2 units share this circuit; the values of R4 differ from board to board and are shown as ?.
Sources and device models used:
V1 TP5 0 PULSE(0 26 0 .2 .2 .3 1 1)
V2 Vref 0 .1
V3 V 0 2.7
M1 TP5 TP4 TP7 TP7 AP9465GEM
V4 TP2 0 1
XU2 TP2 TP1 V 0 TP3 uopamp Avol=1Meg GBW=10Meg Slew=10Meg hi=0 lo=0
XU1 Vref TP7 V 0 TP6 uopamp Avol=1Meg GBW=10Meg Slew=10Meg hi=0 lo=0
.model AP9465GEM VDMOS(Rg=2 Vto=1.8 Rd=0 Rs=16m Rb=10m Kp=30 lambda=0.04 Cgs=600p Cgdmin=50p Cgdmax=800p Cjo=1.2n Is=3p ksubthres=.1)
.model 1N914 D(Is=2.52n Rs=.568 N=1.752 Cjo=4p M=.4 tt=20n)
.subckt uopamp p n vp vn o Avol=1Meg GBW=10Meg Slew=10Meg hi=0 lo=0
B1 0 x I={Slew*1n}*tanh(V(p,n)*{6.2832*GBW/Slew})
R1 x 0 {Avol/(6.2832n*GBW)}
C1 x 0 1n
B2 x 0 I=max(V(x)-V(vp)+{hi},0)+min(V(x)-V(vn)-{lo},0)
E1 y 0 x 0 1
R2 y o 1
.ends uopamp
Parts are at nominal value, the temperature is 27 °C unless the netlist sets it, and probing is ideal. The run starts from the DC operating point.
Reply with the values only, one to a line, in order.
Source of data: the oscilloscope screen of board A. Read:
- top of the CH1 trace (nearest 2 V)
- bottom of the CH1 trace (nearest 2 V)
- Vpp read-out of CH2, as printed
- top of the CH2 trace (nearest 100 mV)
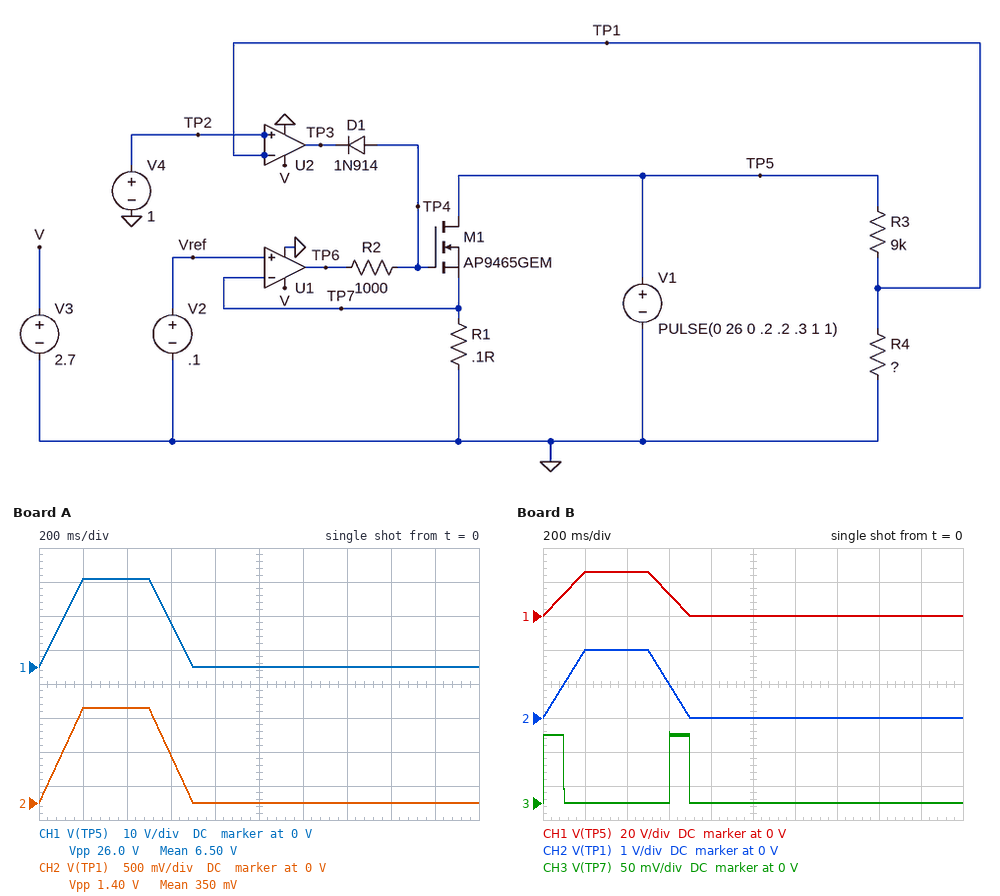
26 V
0 V
1.40 V
1.4 V
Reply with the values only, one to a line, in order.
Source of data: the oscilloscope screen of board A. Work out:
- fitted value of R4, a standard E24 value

510 Ω
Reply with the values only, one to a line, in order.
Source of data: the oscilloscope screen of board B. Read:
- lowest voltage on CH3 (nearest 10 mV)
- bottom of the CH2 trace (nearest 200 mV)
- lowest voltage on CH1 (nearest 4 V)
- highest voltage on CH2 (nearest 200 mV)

0 V
0 V
0 V
2.0 V
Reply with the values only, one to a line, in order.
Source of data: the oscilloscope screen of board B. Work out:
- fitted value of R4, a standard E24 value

750 Ω
